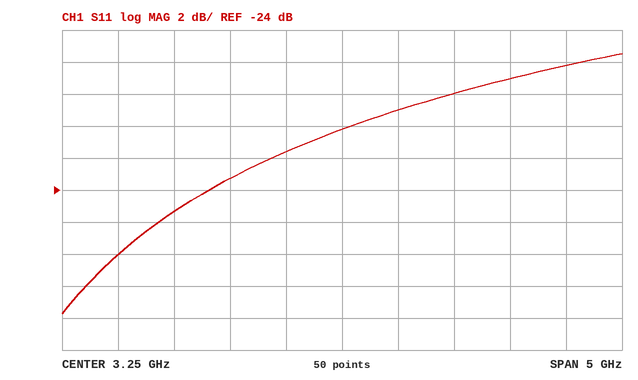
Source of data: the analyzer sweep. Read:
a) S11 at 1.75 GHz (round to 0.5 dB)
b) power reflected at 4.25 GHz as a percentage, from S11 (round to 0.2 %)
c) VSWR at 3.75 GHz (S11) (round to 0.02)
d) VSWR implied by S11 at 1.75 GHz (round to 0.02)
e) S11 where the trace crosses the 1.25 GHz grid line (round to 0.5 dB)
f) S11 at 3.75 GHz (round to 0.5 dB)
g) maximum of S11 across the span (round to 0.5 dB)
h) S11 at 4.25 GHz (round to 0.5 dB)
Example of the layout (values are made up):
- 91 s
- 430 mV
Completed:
- -25.5 dB
- 1.6 %
- 1.26
- 1.12
- -28.0 dB
- -19.0 dB
- -15.5 dB
- -18.0 dB
